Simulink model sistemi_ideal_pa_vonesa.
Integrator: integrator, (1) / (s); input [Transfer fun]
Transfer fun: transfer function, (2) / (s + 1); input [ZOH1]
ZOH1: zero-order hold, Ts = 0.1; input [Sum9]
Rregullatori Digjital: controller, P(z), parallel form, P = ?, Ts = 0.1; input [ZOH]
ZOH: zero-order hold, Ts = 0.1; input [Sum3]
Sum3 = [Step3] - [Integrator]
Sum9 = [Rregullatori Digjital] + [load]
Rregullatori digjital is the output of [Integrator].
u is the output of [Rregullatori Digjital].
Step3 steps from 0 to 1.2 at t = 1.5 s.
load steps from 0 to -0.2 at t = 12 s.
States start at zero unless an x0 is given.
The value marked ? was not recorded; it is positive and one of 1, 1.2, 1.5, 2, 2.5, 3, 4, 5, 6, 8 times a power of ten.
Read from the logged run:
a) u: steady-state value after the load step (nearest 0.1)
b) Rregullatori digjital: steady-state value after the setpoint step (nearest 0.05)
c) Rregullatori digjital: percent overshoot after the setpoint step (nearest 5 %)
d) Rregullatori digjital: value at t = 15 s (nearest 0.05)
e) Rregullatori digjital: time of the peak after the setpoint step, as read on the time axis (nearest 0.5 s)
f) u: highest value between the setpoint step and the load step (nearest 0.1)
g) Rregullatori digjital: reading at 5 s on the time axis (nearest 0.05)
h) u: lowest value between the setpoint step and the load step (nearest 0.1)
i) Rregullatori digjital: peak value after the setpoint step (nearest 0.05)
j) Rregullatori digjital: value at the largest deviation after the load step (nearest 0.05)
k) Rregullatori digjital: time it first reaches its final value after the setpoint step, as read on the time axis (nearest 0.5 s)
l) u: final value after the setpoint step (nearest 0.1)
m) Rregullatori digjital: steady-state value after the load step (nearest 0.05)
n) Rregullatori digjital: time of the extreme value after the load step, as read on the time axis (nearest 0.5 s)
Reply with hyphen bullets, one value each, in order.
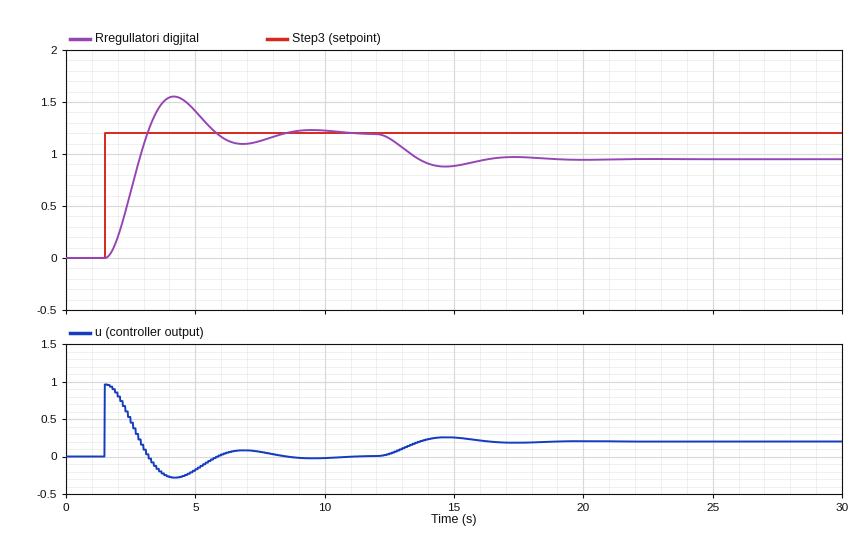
- 0.2
- 1.20
- 30 %
- 0.90
- 4.0 s
- 1.0
- 1.40
- -0.3
- 1.55
- 0.90
- 3.0 s
- 0.0
- 0.95
- 14.5 s
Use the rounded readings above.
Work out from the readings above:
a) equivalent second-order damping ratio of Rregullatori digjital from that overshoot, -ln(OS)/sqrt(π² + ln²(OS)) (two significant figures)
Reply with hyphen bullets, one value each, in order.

- 0.36
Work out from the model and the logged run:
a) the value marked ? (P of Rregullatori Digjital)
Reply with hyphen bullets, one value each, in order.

- 0.8
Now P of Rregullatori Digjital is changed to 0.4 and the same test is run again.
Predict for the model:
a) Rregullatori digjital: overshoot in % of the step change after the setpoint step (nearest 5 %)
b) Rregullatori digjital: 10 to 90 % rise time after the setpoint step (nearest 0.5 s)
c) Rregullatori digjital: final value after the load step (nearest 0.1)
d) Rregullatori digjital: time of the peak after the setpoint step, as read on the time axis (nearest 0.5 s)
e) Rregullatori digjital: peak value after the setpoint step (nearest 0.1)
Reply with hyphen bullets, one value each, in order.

- 15 %
- 2.0 s
- 0.7
- 5.5 s
- 1.4
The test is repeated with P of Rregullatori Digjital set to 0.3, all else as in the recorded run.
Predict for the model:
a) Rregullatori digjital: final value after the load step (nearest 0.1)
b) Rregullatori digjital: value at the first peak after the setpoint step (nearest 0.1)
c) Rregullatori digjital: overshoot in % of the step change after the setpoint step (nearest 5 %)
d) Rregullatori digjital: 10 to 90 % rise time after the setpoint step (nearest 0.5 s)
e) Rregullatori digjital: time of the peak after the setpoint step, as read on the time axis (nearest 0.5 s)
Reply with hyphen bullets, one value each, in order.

- 0.5
- 1.3
- 10 %
- 2.5 s
- 6.5 s
